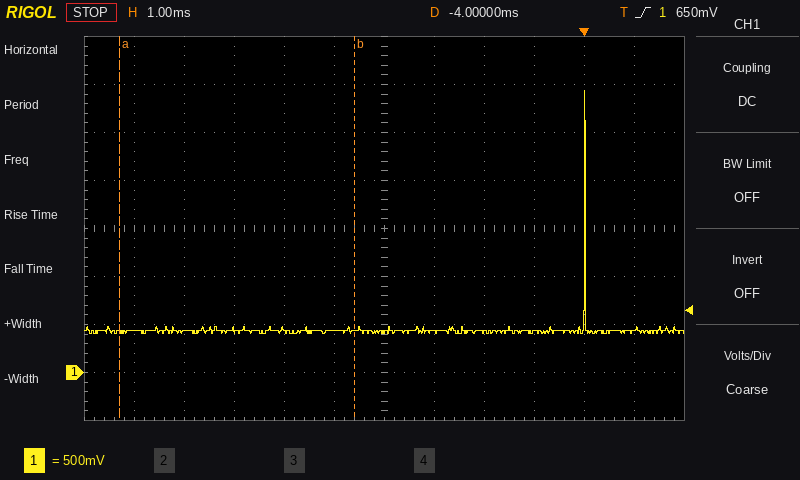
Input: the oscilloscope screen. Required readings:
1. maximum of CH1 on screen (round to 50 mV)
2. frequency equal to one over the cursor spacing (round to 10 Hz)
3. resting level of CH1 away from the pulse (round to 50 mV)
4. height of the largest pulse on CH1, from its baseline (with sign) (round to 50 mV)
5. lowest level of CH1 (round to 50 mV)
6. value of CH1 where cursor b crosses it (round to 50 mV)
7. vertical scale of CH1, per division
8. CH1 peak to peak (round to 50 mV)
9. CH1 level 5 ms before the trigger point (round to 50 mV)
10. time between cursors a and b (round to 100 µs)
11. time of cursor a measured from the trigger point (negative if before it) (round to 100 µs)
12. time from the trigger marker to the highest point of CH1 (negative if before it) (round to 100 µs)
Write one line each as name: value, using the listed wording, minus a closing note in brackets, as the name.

maximum of CH1 on screen: 2.95 V
frequency equal to one over the cursor spacing: 210 Hz
resting level of CH1 away from the pulse: 450 mV
height of the largest pulse on CH1, from its baseline (with sign): +2.50 V
lowest level of CH1: 400 mV
value of CH1 where cursor b crosses it: 450 mV
vertical scale of CH1, per division: 500 mV
CH1 peak to peak: 2.55 V
CH1 level 5 ms before the trigger point: 450 mV
time between cursors a and b: 4.7 ms
time of cursor a measured from the trigger point (negative if before it): -9.3 ms
time from the trigger marker to the highest point of CH1 (negative if before it): 0.0 ms
